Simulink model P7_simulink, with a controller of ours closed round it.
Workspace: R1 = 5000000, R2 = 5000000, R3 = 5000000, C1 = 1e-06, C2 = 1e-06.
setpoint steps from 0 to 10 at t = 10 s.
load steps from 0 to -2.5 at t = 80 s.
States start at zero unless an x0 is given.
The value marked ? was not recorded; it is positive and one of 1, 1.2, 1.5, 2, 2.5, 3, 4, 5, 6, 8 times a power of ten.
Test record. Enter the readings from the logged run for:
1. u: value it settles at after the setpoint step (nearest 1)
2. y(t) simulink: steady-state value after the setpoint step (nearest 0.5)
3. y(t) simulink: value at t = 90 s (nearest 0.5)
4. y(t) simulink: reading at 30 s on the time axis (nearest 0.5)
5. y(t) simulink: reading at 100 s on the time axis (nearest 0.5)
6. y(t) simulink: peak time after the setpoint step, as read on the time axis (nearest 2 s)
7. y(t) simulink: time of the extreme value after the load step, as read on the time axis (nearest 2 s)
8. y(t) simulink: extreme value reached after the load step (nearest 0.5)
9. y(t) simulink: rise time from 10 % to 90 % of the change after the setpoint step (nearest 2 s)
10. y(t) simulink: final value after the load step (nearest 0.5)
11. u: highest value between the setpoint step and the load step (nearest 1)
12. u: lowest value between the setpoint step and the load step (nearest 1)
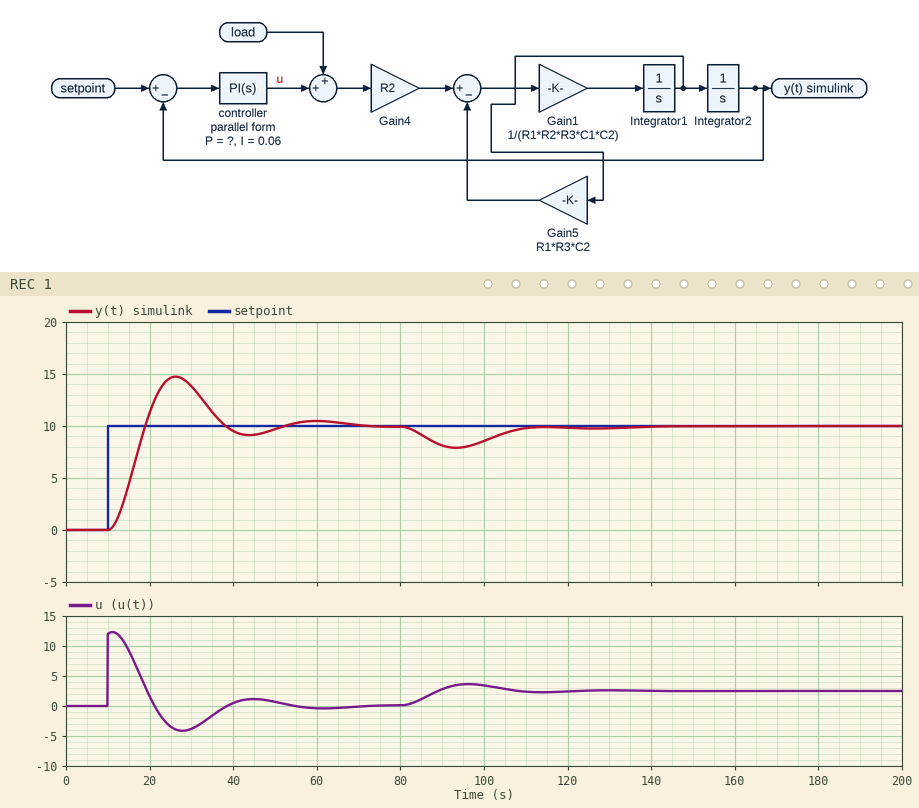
0
10.0
8.0
14.0
8.5
26 s
94 s
8.0
6 s
10.0
12
-4
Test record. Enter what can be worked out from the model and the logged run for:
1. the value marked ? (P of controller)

1.2
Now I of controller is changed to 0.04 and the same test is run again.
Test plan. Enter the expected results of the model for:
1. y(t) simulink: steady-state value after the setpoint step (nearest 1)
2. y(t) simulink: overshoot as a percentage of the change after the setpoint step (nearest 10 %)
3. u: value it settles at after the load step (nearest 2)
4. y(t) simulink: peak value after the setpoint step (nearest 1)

10
40 %
2
14
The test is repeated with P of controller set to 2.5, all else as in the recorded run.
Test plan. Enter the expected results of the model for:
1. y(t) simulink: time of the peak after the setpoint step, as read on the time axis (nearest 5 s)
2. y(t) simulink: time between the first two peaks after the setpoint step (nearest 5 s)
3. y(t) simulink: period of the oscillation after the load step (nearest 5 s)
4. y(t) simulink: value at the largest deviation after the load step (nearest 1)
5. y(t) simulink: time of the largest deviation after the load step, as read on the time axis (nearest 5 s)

20 s
20 s
20 s
9
90 s
